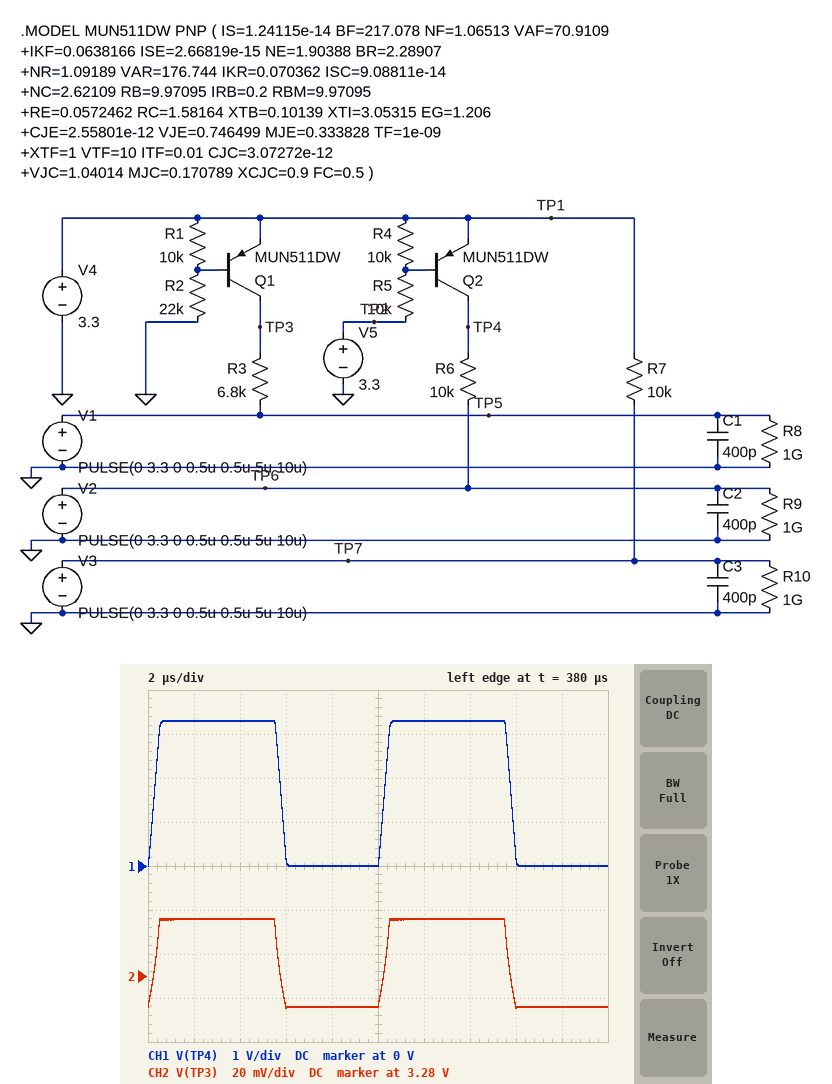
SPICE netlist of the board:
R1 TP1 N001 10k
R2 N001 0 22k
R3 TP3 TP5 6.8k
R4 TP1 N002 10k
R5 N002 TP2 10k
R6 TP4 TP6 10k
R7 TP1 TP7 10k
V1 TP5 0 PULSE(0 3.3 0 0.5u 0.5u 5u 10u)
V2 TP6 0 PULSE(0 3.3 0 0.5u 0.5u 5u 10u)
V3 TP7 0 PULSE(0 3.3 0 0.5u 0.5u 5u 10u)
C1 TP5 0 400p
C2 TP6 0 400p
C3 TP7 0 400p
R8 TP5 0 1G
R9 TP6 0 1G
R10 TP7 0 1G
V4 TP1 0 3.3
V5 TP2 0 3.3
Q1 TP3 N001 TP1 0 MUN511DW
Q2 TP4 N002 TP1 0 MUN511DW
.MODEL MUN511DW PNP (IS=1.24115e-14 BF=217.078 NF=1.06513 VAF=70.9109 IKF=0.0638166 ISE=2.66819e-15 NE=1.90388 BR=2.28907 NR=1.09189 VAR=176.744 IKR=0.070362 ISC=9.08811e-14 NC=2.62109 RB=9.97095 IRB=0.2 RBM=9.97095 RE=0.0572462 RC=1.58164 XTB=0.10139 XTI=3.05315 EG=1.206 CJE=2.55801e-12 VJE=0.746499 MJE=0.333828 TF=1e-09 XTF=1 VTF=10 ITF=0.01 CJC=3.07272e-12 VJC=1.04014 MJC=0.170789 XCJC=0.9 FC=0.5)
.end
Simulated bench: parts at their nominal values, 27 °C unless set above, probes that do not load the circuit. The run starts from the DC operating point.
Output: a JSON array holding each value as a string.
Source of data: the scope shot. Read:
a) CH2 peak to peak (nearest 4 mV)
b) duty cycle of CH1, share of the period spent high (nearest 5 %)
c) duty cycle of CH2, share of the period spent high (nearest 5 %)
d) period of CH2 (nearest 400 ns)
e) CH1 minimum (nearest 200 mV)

["40 mV", "55 %", "55 %", "10.0 µs", "0 V"]
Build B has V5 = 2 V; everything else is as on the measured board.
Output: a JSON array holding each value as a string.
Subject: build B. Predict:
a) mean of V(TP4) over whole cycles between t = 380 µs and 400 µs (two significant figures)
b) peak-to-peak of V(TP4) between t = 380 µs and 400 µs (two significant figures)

["2.8 V", "1.4 V"]
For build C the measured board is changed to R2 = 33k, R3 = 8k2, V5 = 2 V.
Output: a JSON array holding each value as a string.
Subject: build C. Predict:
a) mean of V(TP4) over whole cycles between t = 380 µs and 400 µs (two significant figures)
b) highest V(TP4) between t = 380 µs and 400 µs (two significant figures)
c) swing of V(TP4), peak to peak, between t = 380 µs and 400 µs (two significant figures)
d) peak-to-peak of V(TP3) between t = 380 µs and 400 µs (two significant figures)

["2.8 V", "3.3 V", "1.4 V", "72 mV"]
